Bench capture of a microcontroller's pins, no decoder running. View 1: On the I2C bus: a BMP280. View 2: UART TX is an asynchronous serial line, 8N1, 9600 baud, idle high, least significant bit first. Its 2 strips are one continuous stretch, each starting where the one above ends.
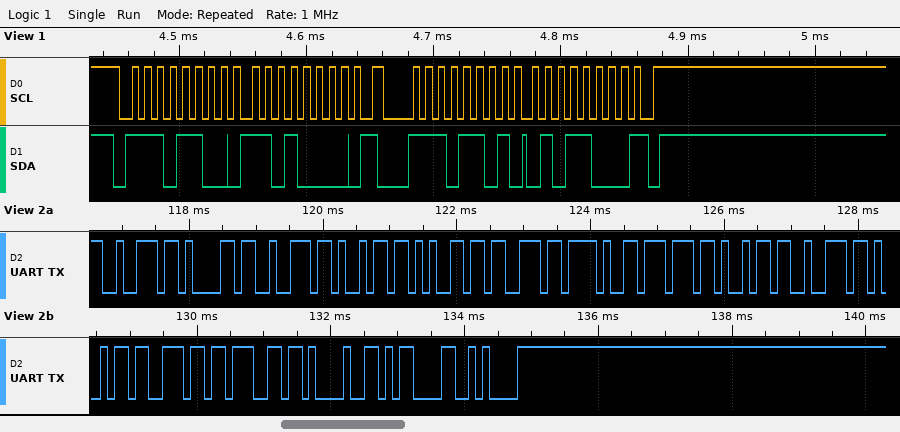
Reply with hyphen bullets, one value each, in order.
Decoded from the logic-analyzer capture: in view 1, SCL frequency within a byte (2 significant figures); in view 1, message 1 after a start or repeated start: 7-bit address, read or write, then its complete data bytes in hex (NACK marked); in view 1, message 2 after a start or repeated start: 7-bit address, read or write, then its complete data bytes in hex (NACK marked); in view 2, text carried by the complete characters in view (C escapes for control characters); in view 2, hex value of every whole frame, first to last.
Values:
- 100 kHz
- 0x76 write: D0
- 0x76 read: 58 NACK
- "raries/wiring!\r\n"
- 0x72 0x61 0x72 0x69 0x65 0x73 0x2F 0x77 0x69 0x72 0x69 0x6E 0x67 0x21 0x0D 0x0A
